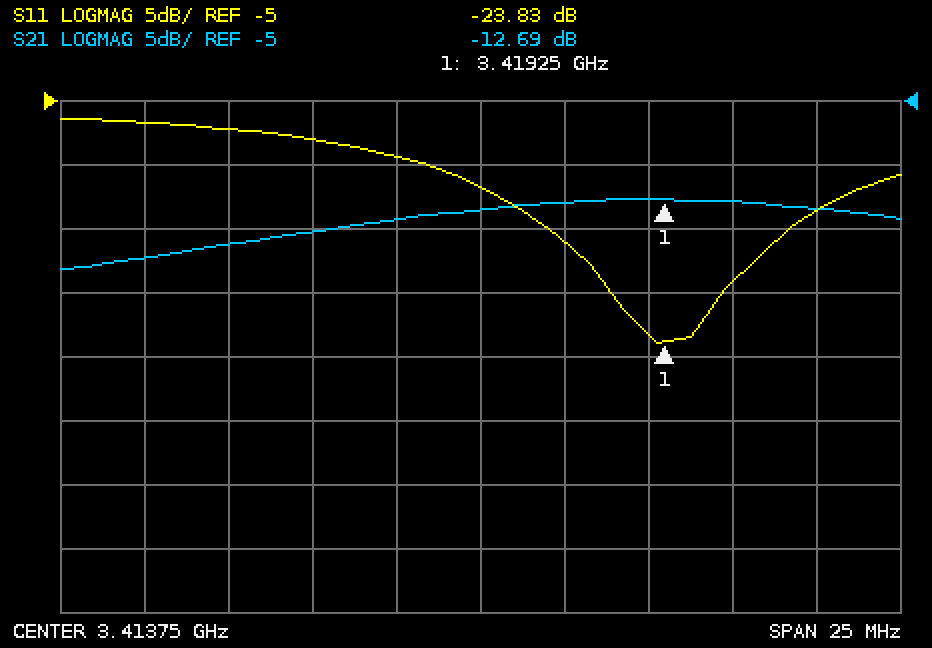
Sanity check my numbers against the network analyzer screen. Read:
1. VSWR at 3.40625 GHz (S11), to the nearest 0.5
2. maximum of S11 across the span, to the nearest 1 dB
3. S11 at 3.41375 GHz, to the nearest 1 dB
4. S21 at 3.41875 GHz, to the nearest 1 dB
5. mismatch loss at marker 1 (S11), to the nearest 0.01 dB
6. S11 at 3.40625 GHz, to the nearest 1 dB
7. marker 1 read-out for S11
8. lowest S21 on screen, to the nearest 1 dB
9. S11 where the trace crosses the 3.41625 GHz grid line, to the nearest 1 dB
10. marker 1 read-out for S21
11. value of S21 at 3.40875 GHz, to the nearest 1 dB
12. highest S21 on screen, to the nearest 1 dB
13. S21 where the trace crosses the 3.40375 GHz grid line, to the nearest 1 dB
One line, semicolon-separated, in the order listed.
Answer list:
2.5; -6 dB; -12 dB; -13 dB; 0.02 dB; -7 dB; -23.83 dB; -18 dB; -16 dB; -12.69 dB; -15 dB; -13 dB; -17 dB
